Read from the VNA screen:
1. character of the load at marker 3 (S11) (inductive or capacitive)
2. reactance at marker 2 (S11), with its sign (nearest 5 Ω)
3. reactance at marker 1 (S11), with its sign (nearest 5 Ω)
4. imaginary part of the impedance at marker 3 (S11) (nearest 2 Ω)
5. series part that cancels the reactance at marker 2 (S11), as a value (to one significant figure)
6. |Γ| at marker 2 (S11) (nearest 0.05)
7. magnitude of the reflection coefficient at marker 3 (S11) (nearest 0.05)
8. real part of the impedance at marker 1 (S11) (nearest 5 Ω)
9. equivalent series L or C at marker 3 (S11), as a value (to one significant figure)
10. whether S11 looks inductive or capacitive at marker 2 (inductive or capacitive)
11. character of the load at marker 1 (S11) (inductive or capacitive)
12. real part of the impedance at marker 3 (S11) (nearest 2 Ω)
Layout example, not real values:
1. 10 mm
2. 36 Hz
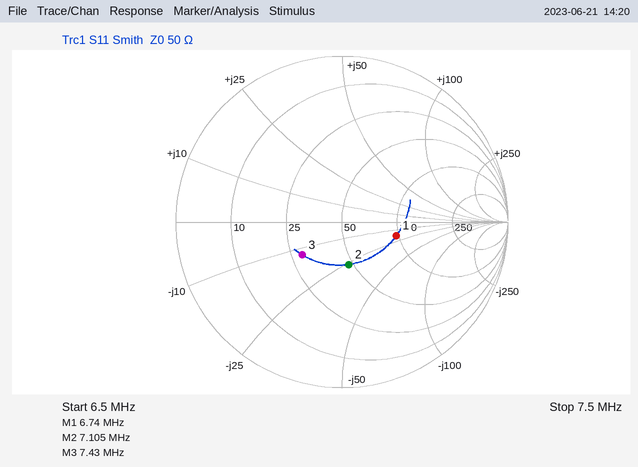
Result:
1. capacitive
2. -25 Ω
3. -20 Ω
4. -12 Ω
5. 600 nH
6. 0.25
7. 0.30
8. 95 Ω
9. 2 nF
10. capacitive
11. capacitive
12. 28 Ω
